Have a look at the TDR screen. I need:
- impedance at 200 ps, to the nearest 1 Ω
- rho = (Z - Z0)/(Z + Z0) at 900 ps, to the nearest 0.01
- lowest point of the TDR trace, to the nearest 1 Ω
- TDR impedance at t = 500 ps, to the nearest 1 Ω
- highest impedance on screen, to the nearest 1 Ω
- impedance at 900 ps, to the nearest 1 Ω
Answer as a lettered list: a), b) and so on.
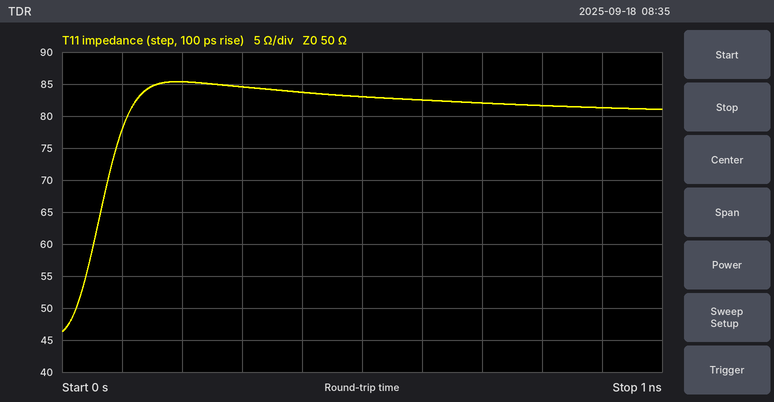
a) 85 Ω
b) +0.24
c) 46 Ω
d) 83 Ω
e) 85 Ω
f) 81 Ω
